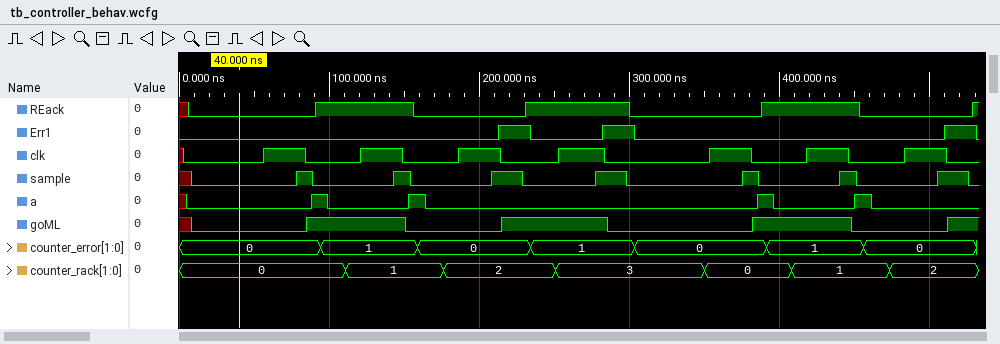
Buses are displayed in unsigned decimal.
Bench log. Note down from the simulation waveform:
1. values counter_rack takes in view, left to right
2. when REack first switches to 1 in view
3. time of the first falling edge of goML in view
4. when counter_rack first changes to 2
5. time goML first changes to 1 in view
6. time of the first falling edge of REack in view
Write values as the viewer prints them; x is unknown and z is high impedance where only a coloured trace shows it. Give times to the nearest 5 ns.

0, 1, 2, 3, 0, 1, 2
90 ns
150 ns
175 ns
85 ns
155 ns
